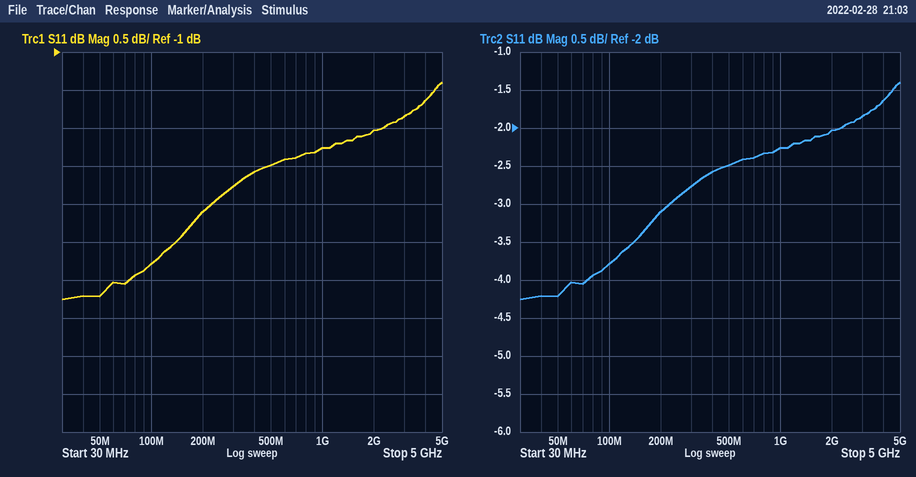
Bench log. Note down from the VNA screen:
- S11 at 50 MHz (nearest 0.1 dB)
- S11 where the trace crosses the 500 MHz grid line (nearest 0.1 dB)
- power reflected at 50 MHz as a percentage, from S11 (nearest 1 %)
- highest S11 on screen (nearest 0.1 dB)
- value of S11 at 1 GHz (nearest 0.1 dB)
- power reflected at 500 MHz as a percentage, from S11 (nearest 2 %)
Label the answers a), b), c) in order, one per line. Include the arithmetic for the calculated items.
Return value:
a) -4.2 dB
b) -2.5 dB
c) 10^(-4.2/10) ≈ 38 %
d) -1.4 dB
e) -2.3 dB
f) 10^(-2.5/10) ≈ 56 %
